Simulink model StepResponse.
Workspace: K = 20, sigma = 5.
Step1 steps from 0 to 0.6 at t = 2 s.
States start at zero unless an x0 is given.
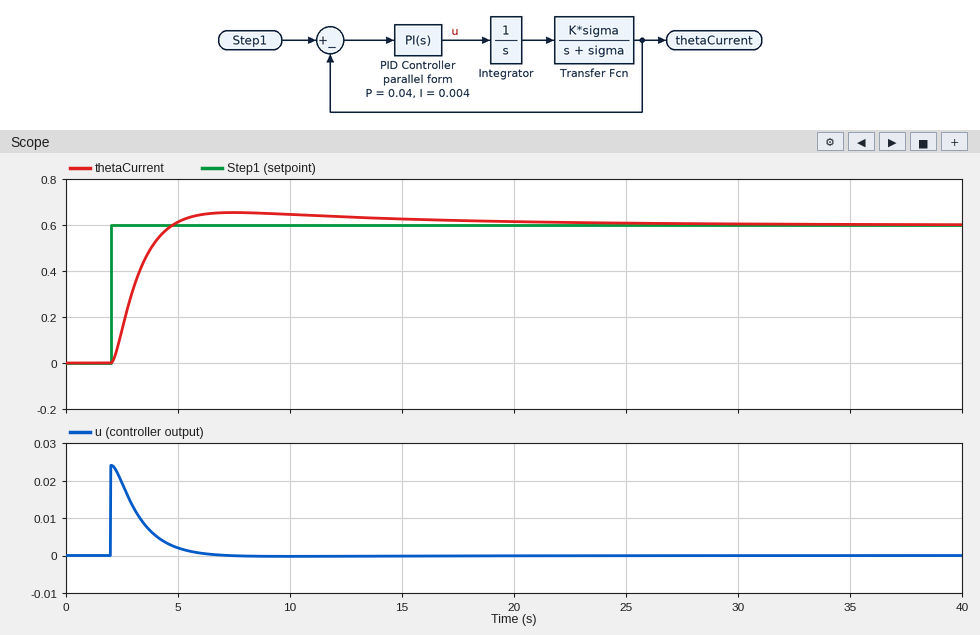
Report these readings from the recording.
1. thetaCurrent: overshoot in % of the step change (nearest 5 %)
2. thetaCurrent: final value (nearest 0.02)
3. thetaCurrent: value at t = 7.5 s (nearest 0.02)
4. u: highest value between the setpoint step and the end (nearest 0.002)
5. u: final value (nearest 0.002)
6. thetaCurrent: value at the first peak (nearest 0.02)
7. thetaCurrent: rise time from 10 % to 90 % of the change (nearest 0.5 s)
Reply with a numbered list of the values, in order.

1. 10 %
2. 0.60
3. 0.66
4. 0.024
5. 0.000
6. 0.66
7. 2.0 s
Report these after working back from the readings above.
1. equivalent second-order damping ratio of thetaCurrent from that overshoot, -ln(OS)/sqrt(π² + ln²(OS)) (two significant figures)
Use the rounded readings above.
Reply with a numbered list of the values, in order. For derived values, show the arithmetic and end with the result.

1. ln(0.1) = -2.303; 2.303 / sqrt(9.870 + 5.302) = 0.59
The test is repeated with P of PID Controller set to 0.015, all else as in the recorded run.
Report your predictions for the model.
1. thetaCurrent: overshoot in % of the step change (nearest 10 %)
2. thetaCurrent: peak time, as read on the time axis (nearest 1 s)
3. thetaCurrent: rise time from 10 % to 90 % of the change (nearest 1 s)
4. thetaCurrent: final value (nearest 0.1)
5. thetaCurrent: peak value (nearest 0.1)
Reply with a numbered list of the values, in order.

1. 30 %
2. 10 s
3. 3 s
4. 0.6
5. 0.8
